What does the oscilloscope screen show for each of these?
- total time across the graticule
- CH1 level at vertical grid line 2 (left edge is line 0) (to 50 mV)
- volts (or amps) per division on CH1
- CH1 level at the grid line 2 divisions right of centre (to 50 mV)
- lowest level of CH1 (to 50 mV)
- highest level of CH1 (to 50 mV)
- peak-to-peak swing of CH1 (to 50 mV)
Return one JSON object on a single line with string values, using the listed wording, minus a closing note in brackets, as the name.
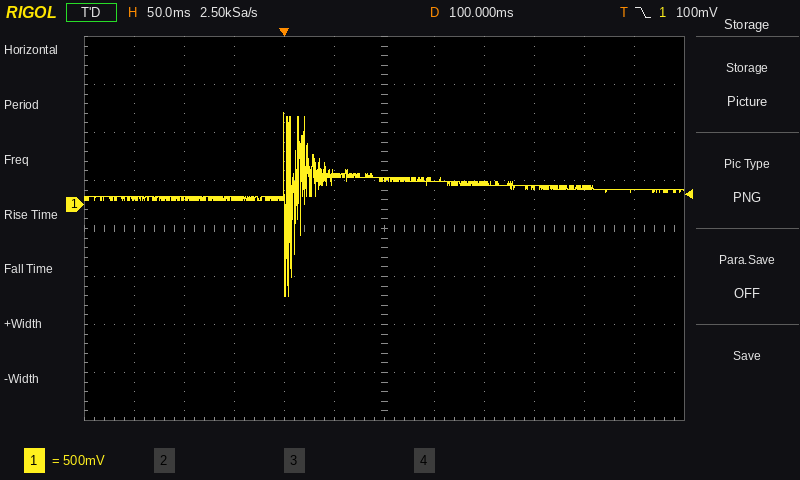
{"total time across the graticule": "600 ms", "CH1 level at vertical grid line 2 (left edge is line 0)": "50 mV", "volts (or amps) per division on CH1": "500 mV", "CH1 level at the grid line 2 divisions right of centre": "200 mV", "lowest level of CH1": "-950 mV", "highest level of CH1": "950 mV", "peak-to-peak swing of CH1": "1.90 V"}
